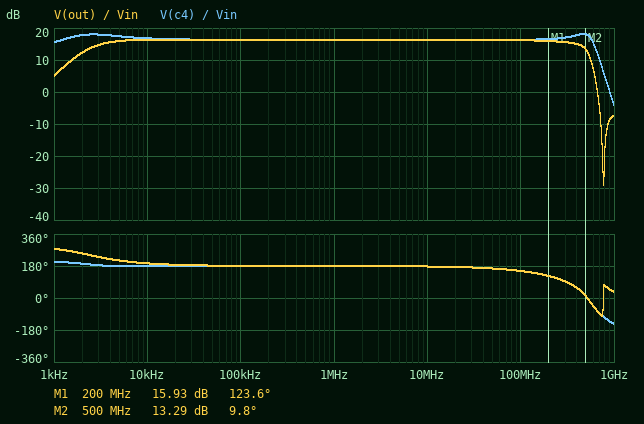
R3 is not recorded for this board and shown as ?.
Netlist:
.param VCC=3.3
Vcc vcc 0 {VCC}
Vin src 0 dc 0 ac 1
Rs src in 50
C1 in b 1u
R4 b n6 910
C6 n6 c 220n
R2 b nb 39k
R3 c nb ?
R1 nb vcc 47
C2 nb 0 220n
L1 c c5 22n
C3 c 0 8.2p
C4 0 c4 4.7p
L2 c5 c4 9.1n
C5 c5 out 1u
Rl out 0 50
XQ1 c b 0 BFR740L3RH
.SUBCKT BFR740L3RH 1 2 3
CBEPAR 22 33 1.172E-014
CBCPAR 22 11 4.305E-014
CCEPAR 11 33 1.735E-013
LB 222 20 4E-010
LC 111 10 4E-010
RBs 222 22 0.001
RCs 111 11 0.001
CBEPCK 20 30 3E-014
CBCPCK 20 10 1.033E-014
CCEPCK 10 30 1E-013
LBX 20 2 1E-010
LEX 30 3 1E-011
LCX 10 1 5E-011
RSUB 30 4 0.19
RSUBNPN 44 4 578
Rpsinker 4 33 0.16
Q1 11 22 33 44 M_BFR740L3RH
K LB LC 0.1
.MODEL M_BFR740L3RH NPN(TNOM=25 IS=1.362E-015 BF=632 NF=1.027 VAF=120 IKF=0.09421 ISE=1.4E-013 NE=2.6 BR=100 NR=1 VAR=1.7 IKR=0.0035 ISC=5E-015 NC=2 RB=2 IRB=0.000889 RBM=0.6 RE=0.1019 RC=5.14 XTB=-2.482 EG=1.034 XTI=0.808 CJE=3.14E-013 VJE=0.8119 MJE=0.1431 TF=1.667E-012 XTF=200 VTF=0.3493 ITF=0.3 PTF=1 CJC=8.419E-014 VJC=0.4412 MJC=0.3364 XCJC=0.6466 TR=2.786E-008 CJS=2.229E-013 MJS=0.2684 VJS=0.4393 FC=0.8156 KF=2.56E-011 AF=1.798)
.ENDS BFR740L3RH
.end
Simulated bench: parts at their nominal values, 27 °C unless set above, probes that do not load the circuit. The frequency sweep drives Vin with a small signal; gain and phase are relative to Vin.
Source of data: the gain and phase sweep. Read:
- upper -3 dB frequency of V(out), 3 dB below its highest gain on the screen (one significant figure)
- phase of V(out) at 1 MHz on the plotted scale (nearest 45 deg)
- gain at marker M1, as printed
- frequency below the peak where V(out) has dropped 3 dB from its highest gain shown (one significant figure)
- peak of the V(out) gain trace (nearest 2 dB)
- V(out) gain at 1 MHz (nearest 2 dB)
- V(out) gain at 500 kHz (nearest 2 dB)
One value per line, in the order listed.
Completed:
500 MHz
180 deg
15.93 dB
2 kHz
16 dB
16 dB
16 dB
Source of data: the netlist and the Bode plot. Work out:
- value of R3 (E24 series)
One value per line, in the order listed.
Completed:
150 Ω
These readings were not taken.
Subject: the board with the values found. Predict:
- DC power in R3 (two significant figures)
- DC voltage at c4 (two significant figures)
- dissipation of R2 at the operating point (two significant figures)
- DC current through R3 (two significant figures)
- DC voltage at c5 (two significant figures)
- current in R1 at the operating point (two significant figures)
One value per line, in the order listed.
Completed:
24 mW
820 mV
92 µW
13 mA
820 mV
13 mA
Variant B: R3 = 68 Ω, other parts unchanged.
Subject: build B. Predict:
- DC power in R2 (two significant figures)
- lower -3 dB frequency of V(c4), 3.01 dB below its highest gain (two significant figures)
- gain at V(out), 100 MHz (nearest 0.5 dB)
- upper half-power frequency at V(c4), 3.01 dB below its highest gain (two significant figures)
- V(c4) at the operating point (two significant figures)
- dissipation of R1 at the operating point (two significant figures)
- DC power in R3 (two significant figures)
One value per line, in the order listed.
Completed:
91 µW
920 Hz
15.0 dB
610 MHz
1.8 V
7.7 mW
11 mW
